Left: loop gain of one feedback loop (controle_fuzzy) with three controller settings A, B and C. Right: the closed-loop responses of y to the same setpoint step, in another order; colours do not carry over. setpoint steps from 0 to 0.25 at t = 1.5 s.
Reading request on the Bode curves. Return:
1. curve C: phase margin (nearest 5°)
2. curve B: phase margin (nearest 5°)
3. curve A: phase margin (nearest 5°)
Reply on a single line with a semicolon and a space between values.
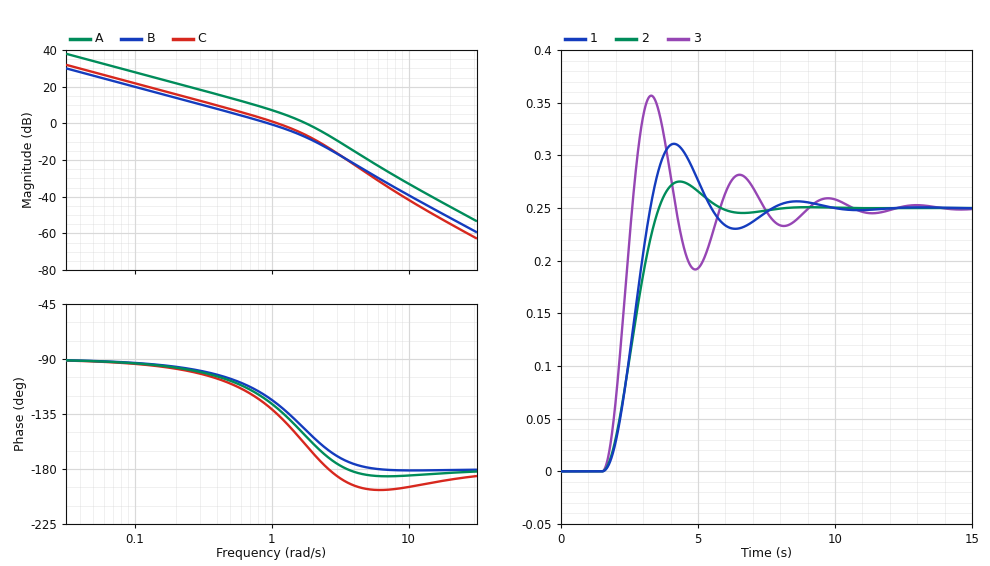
45°; 60°; 25°
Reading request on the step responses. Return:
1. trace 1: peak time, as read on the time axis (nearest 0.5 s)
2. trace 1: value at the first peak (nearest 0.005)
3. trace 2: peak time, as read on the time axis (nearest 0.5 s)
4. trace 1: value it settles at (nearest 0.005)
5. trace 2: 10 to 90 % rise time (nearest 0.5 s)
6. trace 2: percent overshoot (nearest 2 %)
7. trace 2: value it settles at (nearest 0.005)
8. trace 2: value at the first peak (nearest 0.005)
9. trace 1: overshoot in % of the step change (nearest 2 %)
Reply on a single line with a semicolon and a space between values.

4.0 s; 0.310; 4.5 s; 0.250; 1.5 s; 10 %; 0.250; 0.275; 24 %
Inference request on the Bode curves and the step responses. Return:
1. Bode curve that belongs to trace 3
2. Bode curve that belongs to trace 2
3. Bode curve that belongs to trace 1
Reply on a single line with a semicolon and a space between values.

A; B; C
